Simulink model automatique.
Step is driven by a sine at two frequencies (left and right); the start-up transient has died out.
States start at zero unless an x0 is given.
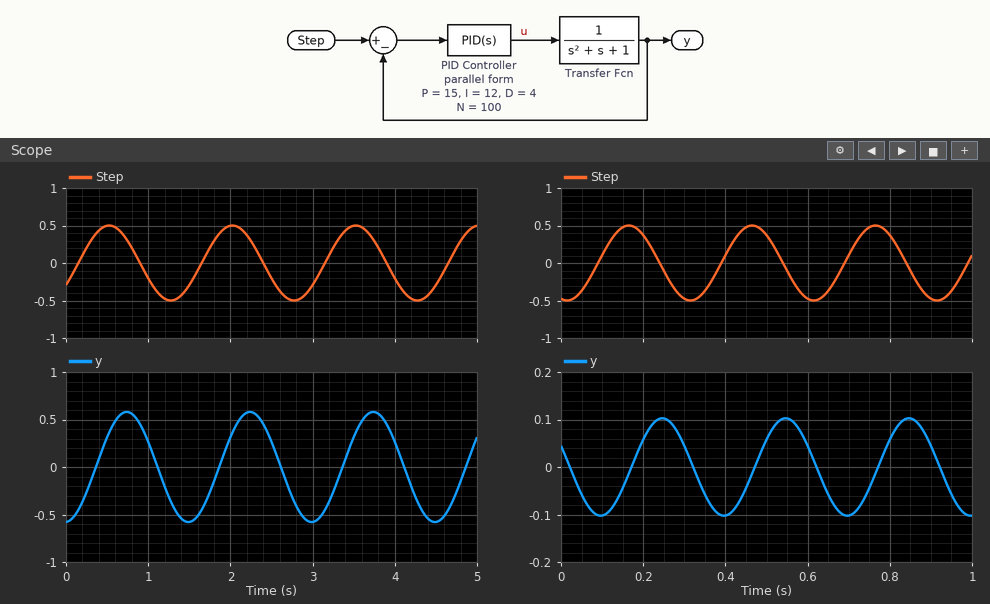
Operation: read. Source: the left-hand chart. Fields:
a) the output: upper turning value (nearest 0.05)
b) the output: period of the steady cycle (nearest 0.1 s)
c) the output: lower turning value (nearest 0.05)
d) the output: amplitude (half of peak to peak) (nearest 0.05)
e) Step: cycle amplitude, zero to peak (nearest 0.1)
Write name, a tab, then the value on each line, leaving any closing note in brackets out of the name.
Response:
the output: upper turning value	0.60
the output: period of the steady cycle	1.5 s
the output: lower turning value	-0.60
the output: amplitude (half of peak to peak)	0.60
Step: cycle amplitude, zero to peak	0.5
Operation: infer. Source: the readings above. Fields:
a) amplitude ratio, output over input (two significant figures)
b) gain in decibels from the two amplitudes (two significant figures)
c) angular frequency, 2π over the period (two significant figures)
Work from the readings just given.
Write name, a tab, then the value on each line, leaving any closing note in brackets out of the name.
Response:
amplitude ratio, output over input	1.2
gain in decibels from the two amplitudes	1.6 dB
angular frequency, 2π over the period	4.2 rad/s
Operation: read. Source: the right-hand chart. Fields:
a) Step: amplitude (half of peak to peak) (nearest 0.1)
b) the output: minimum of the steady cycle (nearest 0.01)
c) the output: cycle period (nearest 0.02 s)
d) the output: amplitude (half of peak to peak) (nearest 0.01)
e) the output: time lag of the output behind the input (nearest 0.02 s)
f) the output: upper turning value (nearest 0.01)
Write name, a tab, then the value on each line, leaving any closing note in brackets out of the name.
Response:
Step: amplitude (half of peak to peak)	0.5
the output: minimum of the steady cycle	-0.10
the output: cycle period	0.30 s
the output: amplitude (half of peak to peak)	0.10
the output: time lag of the output behind the input	0.08 s
the output: upper turning value	0.10
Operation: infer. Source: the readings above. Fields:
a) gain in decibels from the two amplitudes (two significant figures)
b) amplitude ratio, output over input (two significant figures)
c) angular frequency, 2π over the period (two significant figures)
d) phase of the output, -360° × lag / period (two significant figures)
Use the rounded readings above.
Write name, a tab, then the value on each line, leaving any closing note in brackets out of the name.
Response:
gain in decibels from the two amplitudes	-14 dB
amplitude ratio, output over input	0.20
angular frequency, 2π over the period	21 rad/s
phase of the output, -360° × lag / period	-96°
